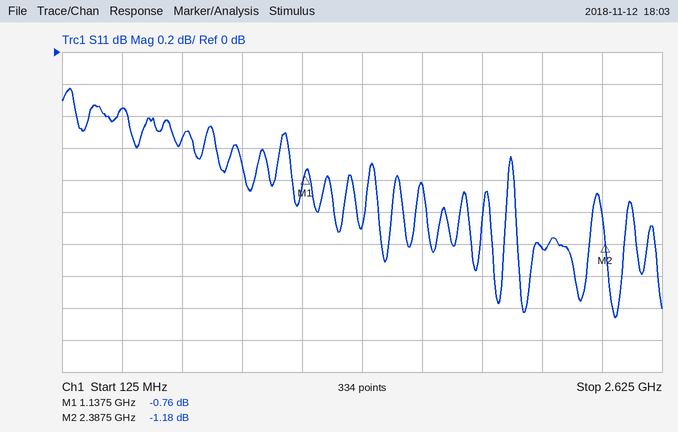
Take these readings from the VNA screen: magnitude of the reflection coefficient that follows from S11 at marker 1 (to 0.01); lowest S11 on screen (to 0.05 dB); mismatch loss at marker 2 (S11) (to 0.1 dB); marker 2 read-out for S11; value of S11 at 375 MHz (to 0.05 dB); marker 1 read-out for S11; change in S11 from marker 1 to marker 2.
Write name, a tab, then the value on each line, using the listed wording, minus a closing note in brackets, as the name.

magnitude of the reflection coefficient that follows from S11 at marker 1	0.92
lowest S11 on screen	-1.65 dB
mismatch loss at marker 2 (S11)	6.2 dB
marker 2 read-out for S11	-1.18 dB
value of S11 at 375 MHz	-0.35 dB
marker 1 read-out for S11	-0.76 dB
change in S11 from marker 1 to marker 2	-0.42 dB
